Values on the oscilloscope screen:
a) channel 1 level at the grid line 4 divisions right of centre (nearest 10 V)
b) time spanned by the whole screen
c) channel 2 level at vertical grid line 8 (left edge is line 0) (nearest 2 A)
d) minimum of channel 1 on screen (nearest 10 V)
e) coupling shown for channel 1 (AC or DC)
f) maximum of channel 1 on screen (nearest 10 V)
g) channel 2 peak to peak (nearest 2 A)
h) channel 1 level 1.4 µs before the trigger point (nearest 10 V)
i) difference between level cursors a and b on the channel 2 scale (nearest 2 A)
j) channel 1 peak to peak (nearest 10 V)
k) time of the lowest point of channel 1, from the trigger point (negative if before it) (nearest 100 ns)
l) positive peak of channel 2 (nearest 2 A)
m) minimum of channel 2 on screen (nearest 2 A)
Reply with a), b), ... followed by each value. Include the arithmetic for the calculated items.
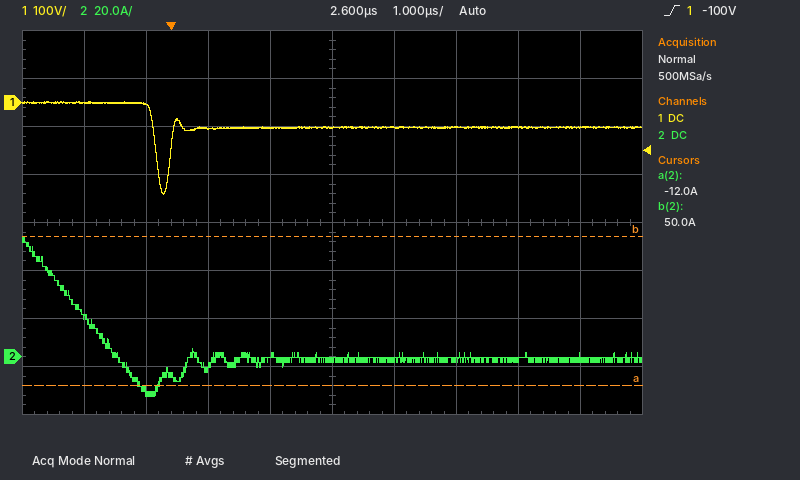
a) -50 V
b) 10 µs
c) -2 A
d) -190 V
e) DC
f) 0 V
g) 50 A − (-16 A) = 66 A
h) 0 V
i) 62 A
j) 0 V − (-190 V) = 190 V
k) -100 ns
l) 50 A
m) -16 A
